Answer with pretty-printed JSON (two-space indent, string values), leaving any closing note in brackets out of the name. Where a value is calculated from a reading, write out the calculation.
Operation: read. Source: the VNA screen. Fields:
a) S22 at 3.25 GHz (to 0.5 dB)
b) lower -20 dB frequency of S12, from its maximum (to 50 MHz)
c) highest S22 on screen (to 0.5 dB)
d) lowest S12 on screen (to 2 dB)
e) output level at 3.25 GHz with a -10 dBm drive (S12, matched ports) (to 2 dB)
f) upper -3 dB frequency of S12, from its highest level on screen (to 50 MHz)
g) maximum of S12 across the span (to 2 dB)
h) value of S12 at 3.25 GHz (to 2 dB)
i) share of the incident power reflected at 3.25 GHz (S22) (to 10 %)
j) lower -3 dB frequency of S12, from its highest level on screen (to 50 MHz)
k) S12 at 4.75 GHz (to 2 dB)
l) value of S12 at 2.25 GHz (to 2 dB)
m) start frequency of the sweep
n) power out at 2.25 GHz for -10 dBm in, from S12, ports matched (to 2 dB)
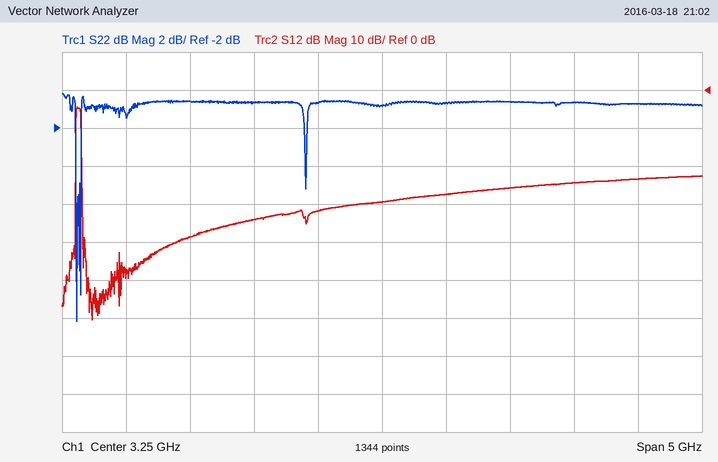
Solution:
{
  "S22 at 3.25 GHz": "-1.0 dB",
  "lower -20 dB frequency of S12, from its maximum": "850 MHz",
  "highest S22 on screen": "0.0 dB",
  "lowest S12 on screen": "-60 dB",
  "output level at 3.25 GHz with a -10 dBm drive (S12, matched ports)": "-10 dBm + (-30 dB) = -40 dBm",
  "upper -3 dB frequency of S12, from its highest level on screen": "900 MHz",
  "maximum of S12 across the span": "-4 dB",
  "value of S12 at 3.25 GHz": "-30 dB",
  "share of the incident power reflected at 3.25 GHz (S22)": "10^(-1/10) ≈ 79.4 %, so 80 % to the nearest 10 %",
  "lower -3 dB frequency of S12, from its highest level on screen": "850 MHz",
  "S12 at 4.75 GHz": "-24 dB",
  "value of S12 at 2.25 GHz": "-34 dB",
  "start frequency of the sweep": "750 MHz",
  "power out at 2.25 GHz for -10 dBm in, from S12, ports matched": "-10 dBm + (-34 dB) = -44 dBm"
}
